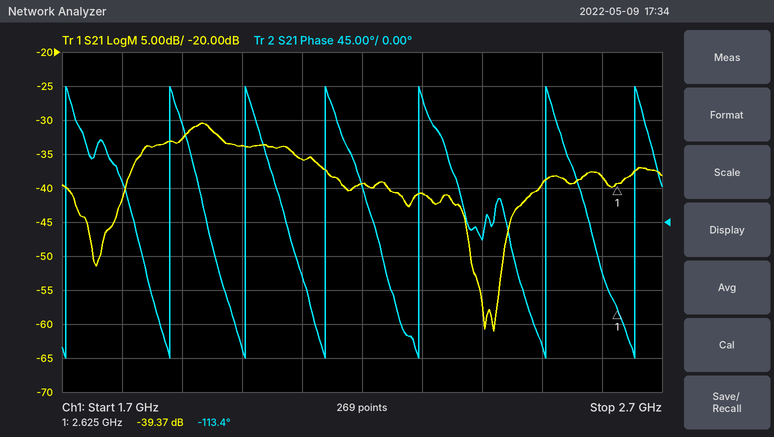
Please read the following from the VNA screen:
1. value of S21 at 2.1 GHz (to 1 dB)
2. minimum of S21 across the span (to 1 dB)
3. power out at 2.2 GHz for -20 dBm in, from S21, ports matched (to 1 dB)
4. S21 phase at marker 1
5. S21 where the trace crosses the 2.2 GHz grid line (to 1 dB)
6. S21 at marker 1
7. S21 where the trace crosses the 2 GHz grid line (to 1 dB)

-36 dB
-61 dB
-59 dBm
-113.4°
-39 dB
-39.37 dB
-34 dB
